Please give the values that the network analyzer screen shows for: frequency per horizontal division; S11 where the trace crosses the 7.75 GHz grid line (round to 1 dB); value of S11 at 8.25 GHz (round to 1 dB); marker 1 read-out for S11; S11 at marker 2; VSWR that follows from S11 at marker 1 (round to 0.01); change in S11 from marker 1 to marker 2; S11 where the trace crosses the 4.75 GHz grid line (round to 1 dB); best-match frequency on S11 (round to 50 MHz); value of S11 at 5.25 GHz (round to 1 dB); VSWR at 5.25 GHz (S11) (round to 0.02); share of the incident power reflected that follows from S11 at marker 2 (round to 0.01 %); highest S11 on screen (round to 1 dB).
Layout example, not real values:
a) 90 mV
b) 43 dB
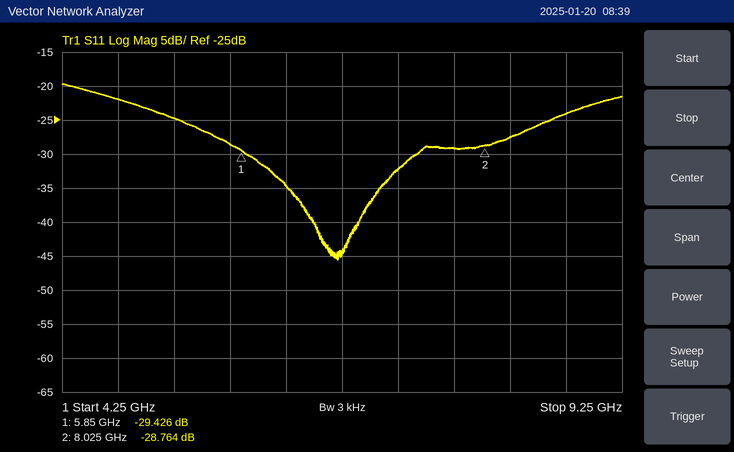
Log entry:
a) 500 MHz
b) -29 dB
c) -28 dB
d) -29.426 dB
e) -28.764 dB
f) 1.07
g) 0.662 dB
h) -22 dB
i) 6.70 GHz
j) -25 dB
k) 1.12
l) 0.13 %
m) -20 dB
